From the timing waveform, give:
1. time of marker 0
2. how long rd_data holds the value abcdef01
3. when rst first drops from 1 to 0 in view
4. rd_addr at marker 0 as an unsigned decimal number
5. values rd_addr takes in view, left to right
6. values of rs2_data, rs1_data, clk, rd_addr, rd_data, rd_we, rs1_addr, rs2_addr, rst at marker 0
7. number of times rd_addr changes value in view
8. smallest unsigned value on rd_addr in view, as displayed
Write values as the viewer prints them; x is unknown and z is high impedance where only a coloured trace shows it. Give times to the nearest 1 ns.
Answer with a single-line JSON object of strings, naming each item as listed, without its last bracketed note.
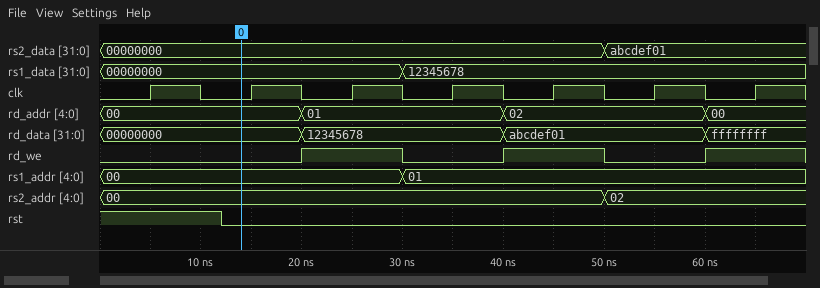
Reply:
{"time of marker 0": "14 ns", "how long rd_data holds the value abcdef01": "20 ns", "when rst first drops from 1 to 0 in view": "12 ns", "rd_addr at marker 0 as an unsigned decimal number": "0", "values rd_addr takes in view, left to right": "00, 01, 02, 00", "values of rs2_data, rs1_data, clk, rd_addr, rd_data, rd_we, rs1_addr, rs2_addr, rst at marker 0": "rs2_data=00000000, rs1_data=00000000, clk=0, rd_addr=00, rd_data=00000000, rd_we=0, rs1_addr=00, rs2_addr=00, rst=0", "number of times rd_addr changes value in view": "3", "smallest unsigned value on rd_addr in view, as displayed": "00"}
